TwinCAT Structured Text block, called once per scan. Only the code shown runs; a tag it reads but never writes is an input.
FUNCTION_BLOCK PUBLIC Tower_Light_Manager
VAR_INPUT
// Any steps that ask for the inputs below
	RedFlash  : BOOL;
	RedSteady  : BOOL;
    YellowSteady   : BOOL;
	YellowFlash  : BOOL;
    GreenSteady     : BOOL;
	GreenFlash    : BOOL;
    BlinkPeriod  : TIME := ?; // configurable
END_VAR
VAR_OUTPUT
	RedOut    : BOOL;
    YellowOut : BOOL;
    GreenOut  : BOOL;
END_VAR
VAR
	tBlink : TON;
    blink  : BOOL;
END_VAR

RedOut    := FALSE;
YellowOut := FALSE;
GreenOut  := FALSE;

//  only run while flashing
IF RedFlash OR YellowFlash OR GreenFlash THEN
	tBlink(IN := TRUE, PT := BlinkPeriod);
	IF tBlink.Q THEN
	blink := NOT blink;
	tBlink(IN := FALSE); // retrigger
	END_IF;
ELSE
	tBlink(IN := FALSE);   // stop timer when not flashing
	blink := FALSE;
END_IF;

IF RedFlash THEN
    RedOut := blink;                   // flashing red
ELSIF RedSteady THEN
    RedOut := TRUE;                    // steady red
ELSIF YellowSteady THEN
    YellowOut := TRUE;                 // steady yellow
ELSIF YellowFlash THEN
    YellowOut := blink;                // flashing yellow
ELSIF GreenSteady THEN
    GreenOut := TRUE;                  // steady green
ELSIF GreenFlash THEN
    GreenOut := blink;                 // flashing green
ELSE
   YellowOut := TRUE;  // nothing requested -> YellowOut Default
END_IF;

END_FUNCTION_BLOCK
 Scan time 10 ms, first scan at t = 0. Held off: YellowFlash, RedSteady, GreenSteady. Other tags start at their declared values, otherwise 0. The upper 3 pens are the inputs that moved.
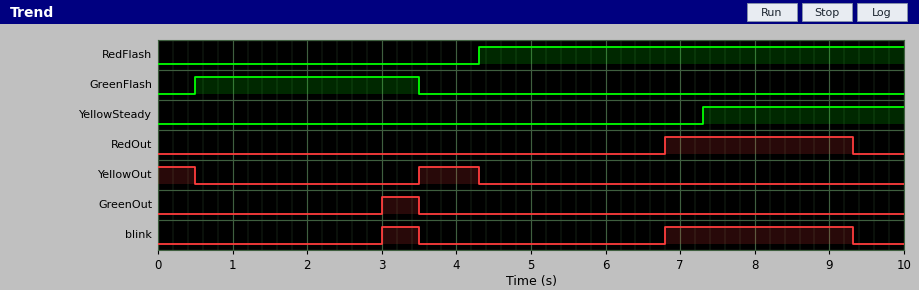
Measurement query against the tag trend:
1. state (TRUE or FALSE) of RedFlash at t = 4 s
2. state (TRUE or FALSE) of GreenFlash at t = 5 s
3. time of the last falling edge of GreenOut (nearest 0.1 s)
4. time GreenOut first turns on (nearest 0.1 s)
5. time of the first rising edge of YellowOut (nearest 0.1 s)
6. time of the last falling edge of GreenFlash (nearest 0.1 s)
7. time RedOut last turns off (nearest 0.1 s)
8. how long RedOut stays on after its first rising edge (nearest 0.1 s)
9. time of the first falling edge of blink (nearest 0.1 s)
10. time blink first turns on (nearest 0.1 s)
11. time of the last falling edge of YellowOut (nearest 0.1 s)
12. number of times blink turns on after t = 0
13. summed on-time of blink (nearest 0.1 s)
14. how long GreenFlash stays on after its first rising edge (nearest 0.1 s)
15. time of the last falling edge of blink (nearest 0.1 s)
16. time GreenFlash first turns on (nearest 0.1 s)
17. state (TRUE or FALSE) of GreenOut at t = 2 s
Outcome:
FALSE
FALSE
3.5 s
3.0 s
3.5 s
3.5 s
9.3 s
2.5 s
3.5 s
3.0 s
4.3 s
2
3.0 s
3.0 s
9.3 s
0.5 s
FALSE
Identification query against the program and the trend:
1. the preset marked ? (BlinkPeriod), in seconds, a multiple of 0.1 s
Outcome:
2.5 s
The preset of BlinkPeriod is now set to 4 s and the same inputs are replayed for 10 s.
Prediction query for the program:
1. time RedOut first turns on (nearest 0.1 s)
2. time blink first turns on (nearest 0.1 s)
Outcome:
8.3 s
8.3 s
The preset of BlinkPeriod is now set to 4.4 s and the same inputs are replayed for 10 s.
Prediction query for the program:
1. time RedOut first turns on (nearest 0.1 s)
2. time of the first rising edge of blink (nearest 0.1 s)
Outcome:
8.7 s
8.7 s
